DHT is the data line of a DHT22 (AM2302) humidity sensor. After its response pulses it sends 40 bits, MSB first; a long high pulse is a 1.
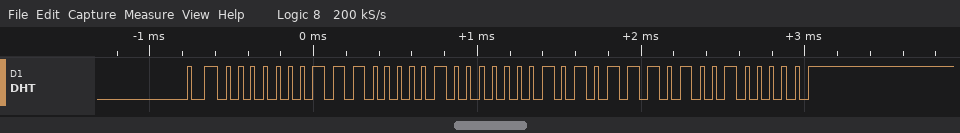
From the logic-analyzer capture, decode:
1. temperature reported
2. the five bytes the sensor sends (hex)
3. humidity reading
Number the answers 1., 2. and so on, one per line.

1. 34.9 °C
2. 01 C1 01 5D 20
3. 44.9 %
